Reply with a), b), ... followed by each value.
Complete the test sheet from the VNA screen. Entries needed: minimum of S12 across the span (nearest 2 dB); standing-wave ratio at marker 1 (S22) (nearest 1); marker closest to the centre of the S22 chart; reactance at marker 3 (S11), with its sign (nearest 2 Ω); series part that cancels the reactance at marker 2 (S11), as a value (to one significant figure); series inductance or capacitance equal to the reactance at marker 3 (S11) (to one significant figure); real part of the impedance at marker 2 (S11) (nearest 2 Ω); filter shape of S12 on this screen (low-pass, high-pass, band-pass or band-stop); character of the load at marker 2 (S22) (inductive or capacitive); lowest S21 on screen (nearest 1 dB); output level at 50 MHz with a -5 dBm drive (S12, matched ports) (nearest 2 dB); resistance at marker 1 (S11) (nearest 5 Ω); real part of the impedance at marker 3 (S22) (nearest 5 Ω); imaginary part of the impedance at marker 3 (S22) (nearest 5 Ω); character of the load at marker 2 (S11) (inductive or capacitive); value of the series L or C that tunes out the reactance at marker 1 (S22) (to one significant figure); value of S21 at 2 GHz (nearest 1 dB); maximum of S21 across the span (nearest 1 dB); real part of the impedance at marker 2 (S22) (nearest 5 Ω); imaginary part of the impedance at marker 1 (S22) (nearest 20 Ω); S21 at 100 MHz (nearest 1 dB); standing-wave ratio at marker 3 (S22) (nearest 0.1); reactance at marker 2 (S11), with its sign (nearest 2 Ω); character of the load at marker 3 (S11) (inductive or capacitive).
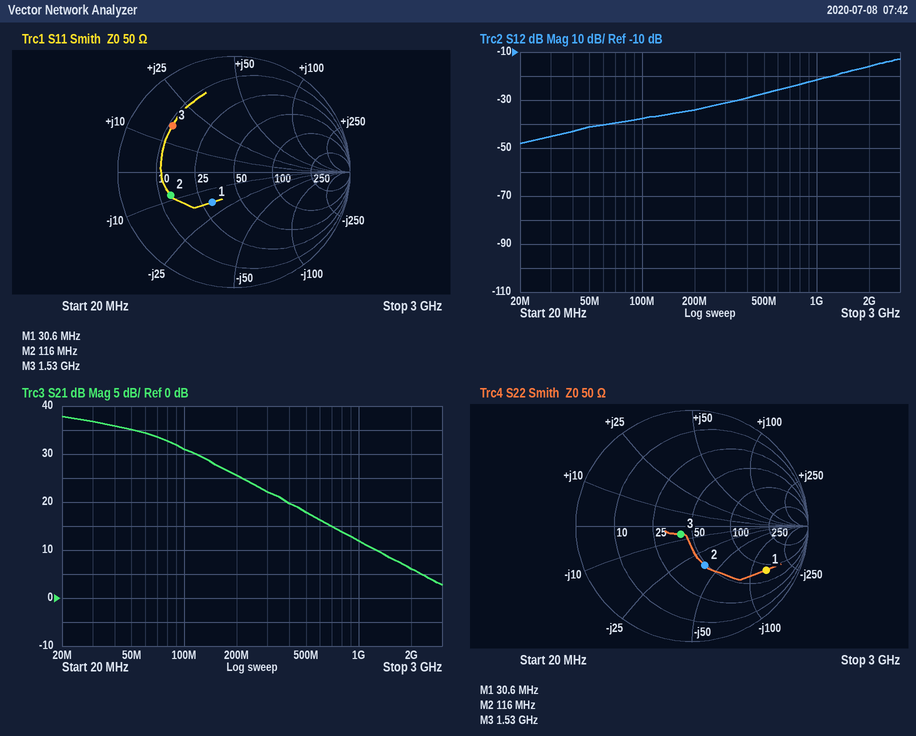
a) -48 dB
b) 7
c) marker 3
d) +16 Ω
e) 10 nH
f) 2 nH
g) 14 Ω
h) high-pass
i) capacitive
j) 3 dB
k) -46 dBm
l) 30 Ω
m) 40 Ω
n) -5 Ω
o) capacitive
p) 700 nH
q) 6 dB
r) 38 dB
s) 50 Ω
t) -140 Ω
u) 31 dB
v) 1.3
w) -8 Ω
x) inductive
